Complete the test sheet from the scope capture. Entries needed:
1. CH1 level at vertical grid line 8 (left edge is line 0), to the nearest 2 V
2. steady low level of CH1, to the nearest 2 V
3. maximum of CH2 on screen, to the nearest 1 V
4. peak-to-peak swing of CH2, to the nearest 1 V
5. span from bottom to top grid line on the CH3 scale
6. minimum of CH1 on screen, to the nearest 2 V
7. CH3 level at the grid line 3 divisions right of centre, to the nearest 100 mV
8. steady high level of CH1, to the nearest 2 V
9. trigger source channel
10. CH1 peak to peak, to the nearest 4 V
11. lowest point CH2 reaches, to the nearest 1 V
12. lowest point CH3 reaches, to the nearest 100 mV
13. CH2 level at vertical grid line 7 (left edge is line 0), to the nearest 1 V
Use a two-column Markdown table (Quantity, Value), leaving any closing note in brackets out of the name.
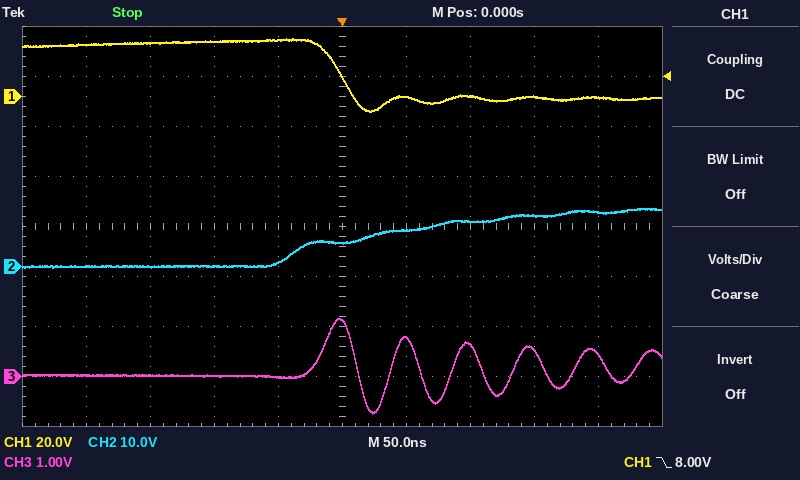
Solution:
| Quantity | Value |
|---|---|
| CH1 level at vertical grid line 8 (left edge is line 0), to the nearest 2 V | 0 V |
| steady low level of CH1, to the nearest 2 V | 0 V |
| maximum of CH2 on screen, to the nearest 1 V | 12 V |
| peak-to-peak swing of CH2, to the nearest 1 V | 12 V |
| span from bottom to top grid line on the CH3 scale | 8 V |
| minimum of CH1 on screen, to the nearest 2 V | -6 V |
| CH3 level at the grid line 3 divisions right of centre, to the nearest 100 mV | 500 mV |
| steady high level of CH1, to the nearest 2 V | 22 V |
| trigger source channel | CH1 |
| CH1 peak to peak, to the nearest 4 V | 28 V |
| lowest point CH2 reaches, to the nearest 1 V | 0 V |
| lowest point CH3 reaches, to the nearest 100 mV | -700 mV |
| CH2 level at vertical grid line 7 (left edge is line 0), to the nearest 1 V | 9 V |
